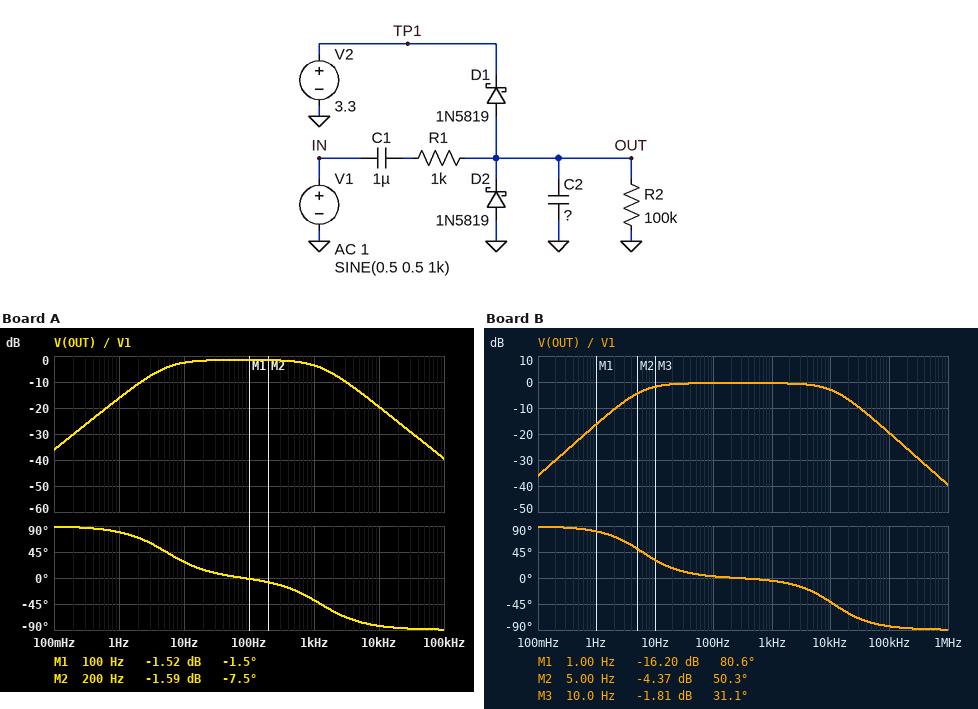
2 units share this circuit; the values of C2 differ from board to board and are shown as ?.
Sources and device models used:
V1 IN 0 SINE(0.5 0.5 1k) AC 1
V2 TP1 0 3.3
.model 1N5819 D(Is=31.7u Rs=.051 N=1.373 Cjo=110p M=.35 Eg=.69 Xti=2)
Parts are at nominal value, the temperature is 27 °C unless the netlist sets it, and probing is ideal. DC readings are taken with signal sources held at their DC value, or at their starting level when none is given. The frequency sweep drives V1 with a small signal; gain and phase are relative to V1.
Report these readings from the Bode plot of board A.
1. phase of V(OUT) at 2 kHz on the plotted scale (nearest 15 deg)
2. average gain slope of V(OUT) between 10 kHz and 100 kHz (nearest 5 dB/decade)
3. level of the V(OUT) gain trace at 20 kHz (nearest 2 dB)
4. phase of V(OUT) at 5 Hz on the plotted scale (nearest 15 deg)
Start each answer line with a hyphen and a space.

- -60 deg
- -20 dB/decade
- -26 dB
- 45 deg
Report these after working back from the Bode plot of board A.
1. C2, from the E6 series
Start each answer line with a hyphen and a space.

- 150 nF
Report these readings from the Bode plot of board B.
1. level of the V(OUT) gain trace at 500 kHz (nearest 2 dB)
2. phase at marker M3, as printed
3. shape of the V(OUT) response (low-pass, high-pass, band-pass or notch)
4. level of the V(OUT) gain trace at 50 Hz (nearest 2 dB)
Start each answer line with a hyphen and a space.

- -34 dB
- 31.1 deg
- band-pass
- 0 dB
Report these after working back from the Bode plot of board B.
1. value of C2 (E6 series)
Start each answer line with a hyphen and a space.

- 15 nF
